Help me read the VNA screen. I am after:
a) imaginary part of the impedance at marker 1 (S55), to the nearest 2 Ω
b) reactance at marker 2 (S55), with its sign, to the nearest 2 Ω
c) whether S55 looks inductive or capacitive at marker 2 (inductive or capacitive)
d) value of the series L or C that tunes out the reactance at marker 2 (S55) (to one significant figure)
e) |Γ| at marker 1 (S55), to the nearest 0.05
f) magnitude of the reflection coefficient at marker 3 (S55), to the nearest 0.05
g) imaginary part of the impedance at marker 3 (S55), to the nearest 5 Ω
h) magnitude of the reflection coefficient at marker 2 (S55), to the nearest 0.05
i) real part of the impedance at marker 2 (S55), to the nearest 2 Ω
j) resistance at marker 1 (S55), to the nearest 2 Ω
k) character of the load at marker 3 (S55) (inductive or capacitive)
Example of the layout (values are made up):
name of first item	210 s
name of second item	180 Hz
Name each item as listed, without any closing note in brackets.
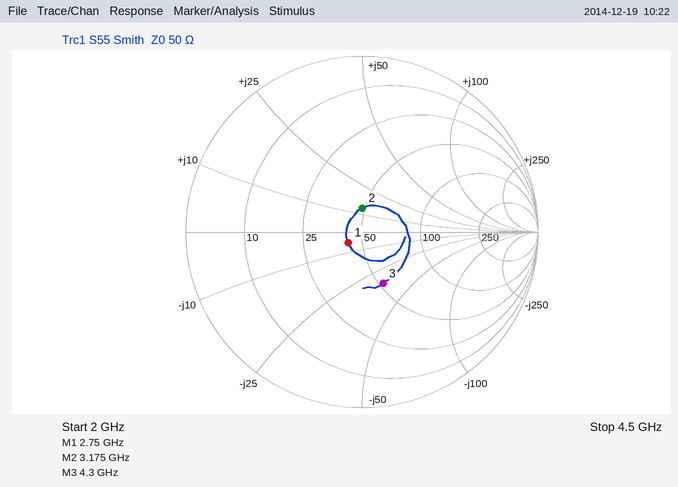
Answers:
imaginary part of the impedance at marker 1 (S55), to the nearest 2 Ω	-6 Ω
reactance at marker 2 (S55), with its sign, to the nearest 2 Ω	+14 Ω
whether S55 looks inductive or capacitive at marker 2	inductive
value of the series L or C that tunes out the reactance at marker 2 (S55)	4 pF
|Γ| at marker 1 (S55), to the nearest 0.05	0.10
magnitude of the reflection coefficient at marker 3 (S55), to the nearest 0.05	0.30
imaginary part of the impedance at marker 3 (S55), to the nearest 5 Ω	-35 Ω
magnitude of the reflection coefficient at marker 2 (S55), to the nearest 0.05	0.15
real part of the impedance at marker 2 (S55), to the nearest 2 Ω	48 Ω
resistance at marker 1 (S55), to the nearest 2 Ω	42 Ω
character of the load at marker 3 (S55)	capacitive
